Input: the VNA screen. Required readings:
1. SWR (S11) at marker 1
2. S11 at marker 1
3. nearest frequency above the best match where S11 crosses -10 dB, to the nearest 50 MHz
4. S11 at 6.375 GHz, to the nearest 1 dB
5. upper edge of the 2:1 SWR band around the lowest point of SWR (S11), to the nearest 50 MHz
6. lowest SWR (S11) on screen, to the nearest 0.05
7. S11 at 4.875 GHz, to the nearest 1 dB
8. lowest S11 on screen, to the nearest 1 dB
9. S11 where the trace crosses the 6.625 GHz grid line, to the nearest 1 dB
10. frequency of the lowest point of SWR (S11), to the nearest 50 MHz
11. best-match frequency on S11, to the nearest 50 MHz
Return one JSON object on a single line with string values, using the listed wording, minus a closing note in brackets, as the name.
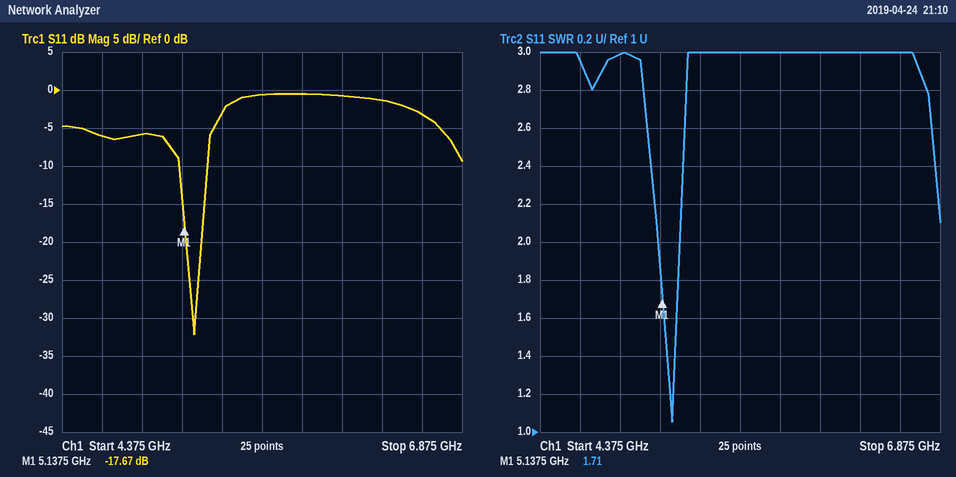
{"SWR (S11) at marker 1": "1.71", "S11 at marker 1": "-17.67 dB", "nearest frequency above the best match where S11 crosses -10 dB, to the nearest 50 MHz": "5.30 GHz", "S11 at 6.375 GHz, to the nearest 1 dB": "-1 dB", "upper edge of the 2:1 SWR band around the lowest point of SWR (S11), to the nearest 50 MHz": "5.25 GHz", "lowest SWR (S11) on screen, to the nearest 0.05": "1.05", "S11 at 4.875 GHz, to the nearest 1 dB": "-6 dB", "lowest S11 on screen, to the nearest 1 dB": "-32 dB", "S11 where the trace crosses the 6.625 GHz grid line, to the nearest 1 dB": "-3 dB", "frequency of the lowest point of SWR (S11), to the nearest 50 MHz": "5.20 GHz", "best-match frequency on S11, to the nearest 50 MHz": "5.20 GHz"}
